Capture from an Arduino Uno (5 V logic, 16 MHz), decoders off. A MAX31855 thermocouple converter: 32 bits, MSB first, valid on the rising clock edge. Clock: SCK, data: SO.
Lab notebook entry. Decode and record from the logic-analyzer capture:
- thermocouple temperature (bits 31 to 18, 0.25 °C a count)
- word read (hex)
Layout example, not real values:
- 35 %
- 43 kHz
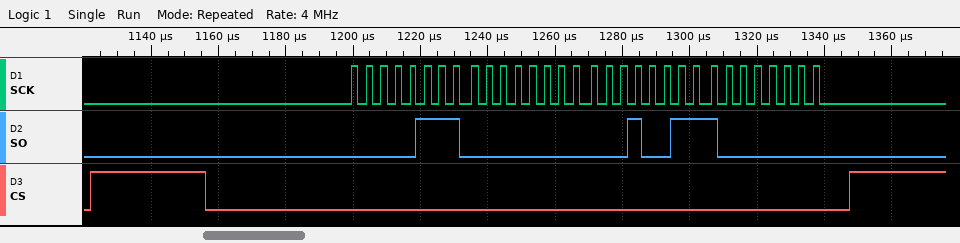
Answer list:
- 112.00 °C
- 0x07001380
